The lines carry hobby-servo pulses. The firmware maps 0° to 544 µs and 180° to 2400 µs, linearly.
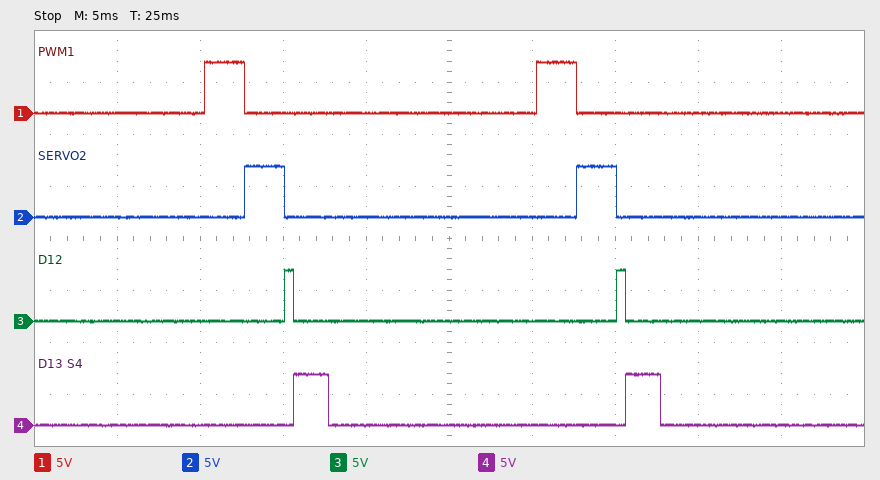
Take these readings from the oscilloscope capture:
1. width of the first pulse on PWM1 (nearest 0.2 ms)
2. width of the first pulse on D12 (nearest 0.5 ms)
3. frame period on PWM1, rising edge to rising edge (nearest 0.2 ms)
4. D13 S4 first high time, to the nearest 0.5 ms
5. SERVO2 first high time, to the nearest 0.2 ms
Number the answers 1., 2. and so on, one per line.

1. 2.4 ms
2. 0.5 ms
3. 20.0 ms
4. 2.0 ms
5. 2.4 ms
